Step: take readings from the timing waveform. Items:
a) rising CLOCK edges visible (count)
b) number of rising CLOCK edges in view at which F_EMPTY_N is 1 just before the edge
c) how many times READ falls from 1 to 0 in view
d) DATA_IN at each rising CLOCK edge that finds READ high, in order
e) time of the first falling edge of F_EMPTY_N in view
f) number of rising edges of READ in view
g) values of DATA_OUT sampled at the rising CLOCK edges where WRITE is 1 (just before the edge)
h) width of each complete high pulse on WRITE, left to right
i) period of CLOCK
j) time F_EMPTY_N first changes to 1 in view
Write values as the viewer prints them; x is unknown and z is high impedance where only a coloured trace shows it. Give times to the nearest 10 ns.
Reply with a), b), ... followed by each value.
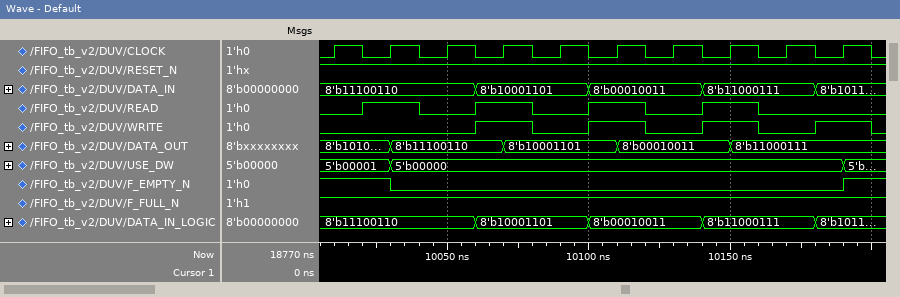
a) 10
b) 2
c) 4
d) 8'b11100110, 8'b10001101, 8'b00010011, 8'b11000111
e) 10030 ns
f) 4
g) 8'b11100110, 8'b10001101, 8'b00010011, 8'b11000111
h) 20 ns, 20 ns, 20 ns, 20 ns
i) 20 ns
j) 10190 ns
